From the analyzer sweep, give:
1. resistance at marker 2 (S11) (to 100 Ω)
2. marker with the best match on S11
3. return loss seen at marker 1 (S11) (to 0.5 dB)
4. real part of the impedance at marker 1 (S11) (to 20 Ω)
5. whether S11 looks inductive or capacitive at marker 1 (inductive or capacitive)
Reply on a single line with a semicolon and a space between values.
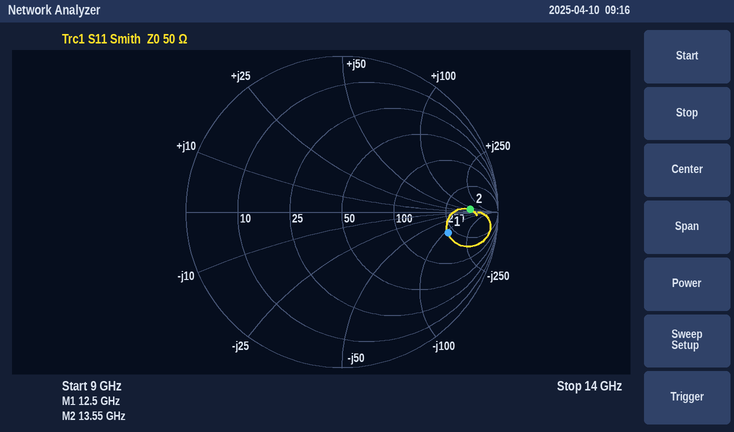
500 Ω; marker 1; 3.0 dB; 220 Ω; capacitive
